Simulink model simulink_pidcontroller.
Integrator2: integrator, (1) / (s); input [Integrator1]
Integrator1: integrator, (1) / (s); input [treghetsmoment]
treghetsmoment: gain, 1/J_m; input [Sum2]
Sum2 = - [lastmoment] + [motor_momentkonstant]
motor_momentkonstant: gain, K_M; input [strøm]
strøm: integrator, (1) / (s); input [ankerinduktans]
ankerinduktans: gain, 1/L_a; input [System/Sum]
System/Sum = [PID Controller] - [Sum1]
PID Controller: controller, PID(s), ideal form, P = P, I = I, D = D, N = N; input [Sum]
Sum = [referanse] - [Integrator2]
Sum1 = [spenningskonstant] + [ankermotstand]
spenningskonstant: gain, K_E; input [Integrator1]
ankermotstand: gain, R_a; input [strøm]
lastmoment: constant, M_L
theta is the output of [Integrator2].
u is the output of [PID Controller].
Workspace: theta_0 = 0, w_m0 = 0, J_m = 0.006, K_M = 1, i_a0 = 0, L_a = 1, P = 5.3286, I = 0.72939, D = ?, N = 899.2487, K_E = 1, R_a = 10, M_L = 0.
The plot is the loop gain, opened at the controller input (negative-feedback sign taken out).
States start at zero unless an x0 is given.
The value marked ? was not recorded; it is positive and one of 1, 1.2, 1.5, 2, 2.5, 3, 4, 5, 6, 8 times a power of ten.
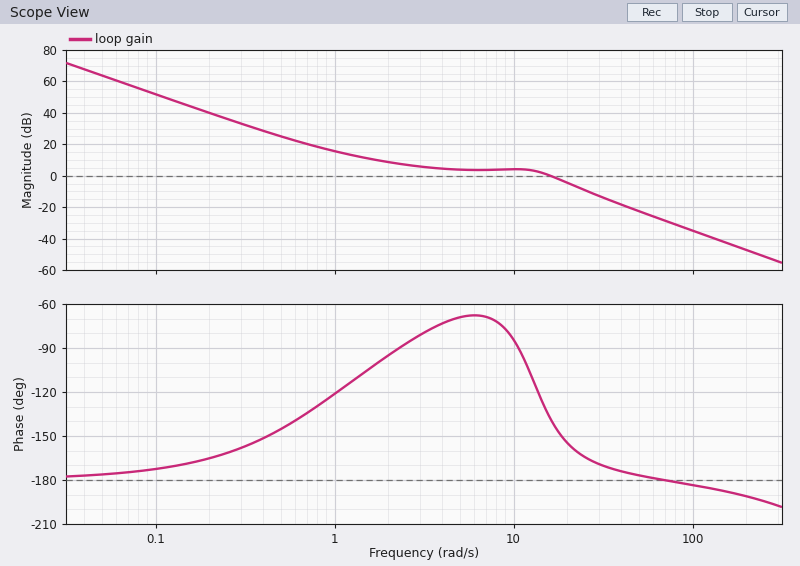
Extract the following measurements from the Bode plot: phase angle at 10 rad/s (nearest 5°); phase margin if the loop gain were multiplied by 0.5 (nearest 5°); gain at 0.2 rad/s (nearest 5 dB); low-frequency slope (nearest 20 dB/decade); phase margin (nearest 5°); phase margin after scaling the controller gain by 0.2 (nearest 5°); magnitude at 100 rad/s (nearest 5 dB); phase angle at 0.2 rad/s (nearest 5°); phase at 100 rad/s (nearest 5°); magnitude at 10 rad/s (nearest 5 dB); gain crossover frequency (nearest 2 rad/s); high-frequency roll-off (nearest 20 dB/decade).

-85°
100°
40 dB
-40 dB/decade
40°
65°
-35 dB
-165°
-185°
5 dB
16 rad/s
-40 dB/decade
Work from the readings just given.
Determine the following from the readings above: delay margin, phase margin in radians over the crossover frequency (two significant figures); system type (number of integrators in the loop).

0.044 s
2
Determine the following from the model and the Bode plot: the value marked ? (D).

0.2
